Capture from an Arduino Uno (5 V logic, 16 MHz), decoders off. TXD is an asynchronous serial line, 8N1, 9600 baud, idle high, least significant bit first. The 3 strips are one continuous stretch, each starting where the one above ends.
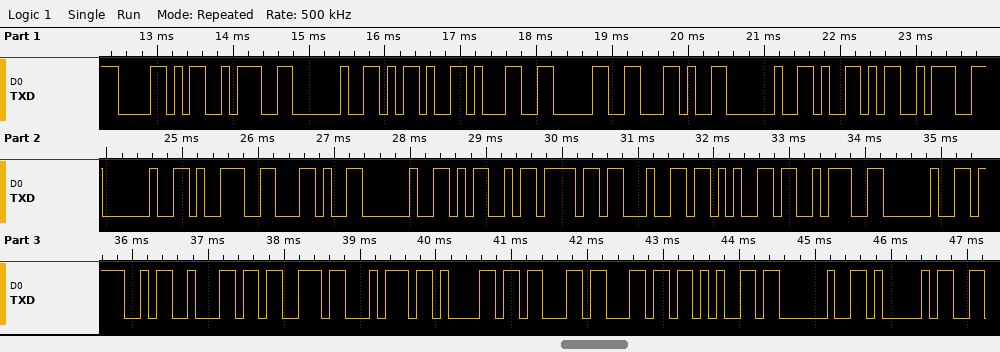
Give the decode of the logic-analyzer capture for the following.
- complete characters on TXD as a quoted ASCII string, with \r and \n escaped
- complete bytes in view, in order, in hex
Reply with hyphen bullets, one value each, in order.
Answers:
- "X: -10, Y: 9, Mode: Obstacle A"
- 58 3A 20 2D 31 30 2C 20 59 3A 20 39 2C 20 4D 6F 64 65 3A 20 4F 62 73 74 61 63 6C 65 20 41
